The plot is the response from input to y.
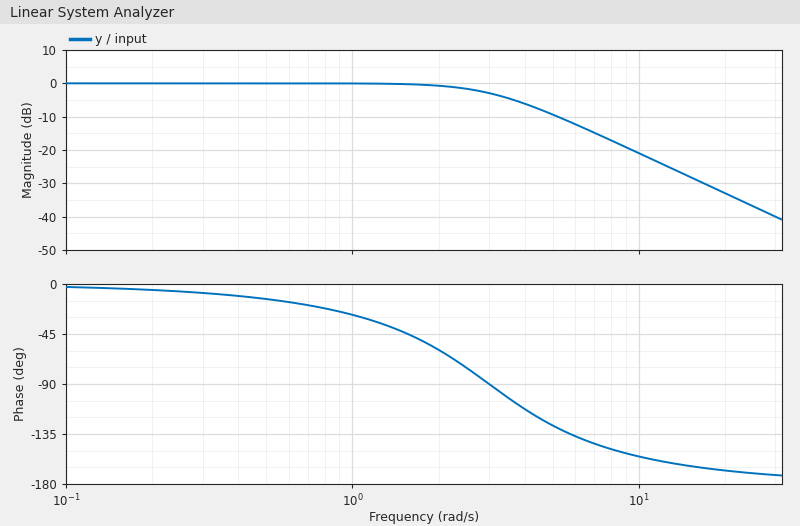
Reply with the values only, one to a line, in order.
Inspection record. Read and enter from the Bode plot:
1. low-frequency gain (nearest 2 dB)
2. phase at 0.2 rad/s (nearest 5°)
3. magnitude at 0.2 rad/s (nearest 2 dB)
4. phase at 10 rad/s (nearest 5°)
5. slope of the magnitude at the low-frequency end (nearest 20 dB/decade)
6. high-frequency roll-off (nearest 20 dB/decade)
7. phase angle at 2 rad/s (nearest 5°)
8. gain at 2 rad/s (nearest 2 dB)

0 dB
-5°
0 dB
-155°
0 dB/decade
-40 dB/decade
-60°
0 dB
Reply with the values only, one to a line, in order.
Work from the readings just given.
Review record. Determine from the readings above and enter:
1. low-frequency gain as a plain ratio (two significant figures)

1.0
